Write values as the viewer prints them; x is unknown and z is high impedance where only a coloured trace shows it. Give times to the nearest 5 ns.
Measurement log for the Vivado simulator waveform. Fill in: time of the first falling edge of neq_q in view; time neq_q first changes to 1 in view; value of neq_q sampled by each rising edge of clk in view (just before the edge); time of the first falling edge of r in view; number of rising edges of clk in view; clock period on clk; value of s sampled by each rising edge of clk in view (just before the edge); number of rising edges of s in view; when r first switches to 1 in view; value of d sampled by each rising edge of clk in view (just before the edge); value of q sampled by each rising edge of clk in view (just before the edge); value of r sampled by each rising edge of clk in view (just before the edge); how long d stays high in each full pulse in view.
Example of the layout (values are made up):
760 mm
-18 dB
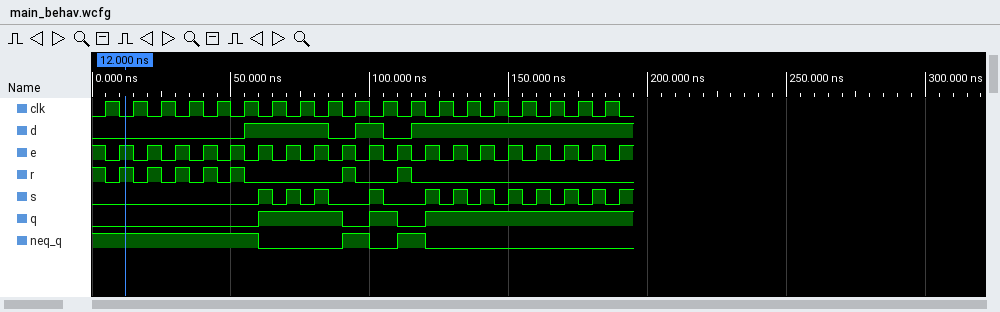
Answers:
60 ns
90 ns
1 1 1 1 1 1 0 0 0 1 0 1 0 0 0 0 0 0 0
5 ns
19
10 ns
0 0 0 0 0 0 1 1 1 0 1 0 1 1 1 1 1 1 1
12
10 ns
0 0 0 0 0 0 1 1 1 0 1 0 1 1 1 1 1 1 1
0 0 0 0 0 0 1 1 1 0 1 0 1 1 1 1 1 1 1
1 1 1 1 1 1 0 0 0 1 0 1 0 0 0 0 0 0 0
30 ns, 10 ns
